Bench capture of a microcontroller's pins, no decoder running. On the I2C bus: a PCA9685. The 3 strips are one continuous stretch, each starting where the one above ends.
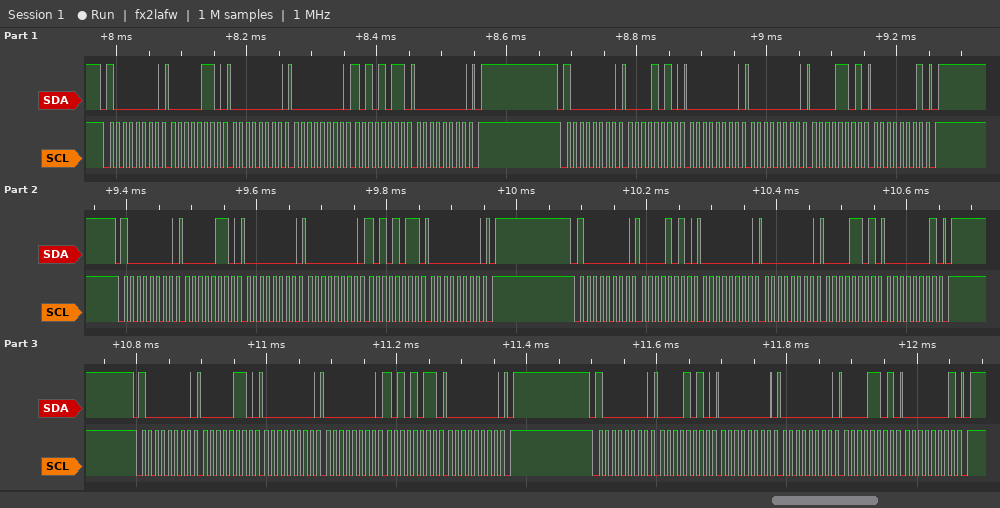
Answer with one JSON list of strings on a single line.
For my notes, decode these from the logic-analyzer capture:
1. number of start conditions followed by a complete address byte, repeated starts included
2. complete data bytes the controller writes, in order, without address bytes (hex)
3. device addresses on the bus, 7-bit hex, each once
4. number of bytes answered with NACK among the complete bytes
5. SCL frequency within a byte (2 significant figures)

["6", "06 00 00 AB 00 0A 00 00 0D 01 06 00 00 AB 00 0A 00 00 0D 01 06 00 00 AB 00 0A 00 00 0D 01", "0x40", "0", "100 kHz"]
